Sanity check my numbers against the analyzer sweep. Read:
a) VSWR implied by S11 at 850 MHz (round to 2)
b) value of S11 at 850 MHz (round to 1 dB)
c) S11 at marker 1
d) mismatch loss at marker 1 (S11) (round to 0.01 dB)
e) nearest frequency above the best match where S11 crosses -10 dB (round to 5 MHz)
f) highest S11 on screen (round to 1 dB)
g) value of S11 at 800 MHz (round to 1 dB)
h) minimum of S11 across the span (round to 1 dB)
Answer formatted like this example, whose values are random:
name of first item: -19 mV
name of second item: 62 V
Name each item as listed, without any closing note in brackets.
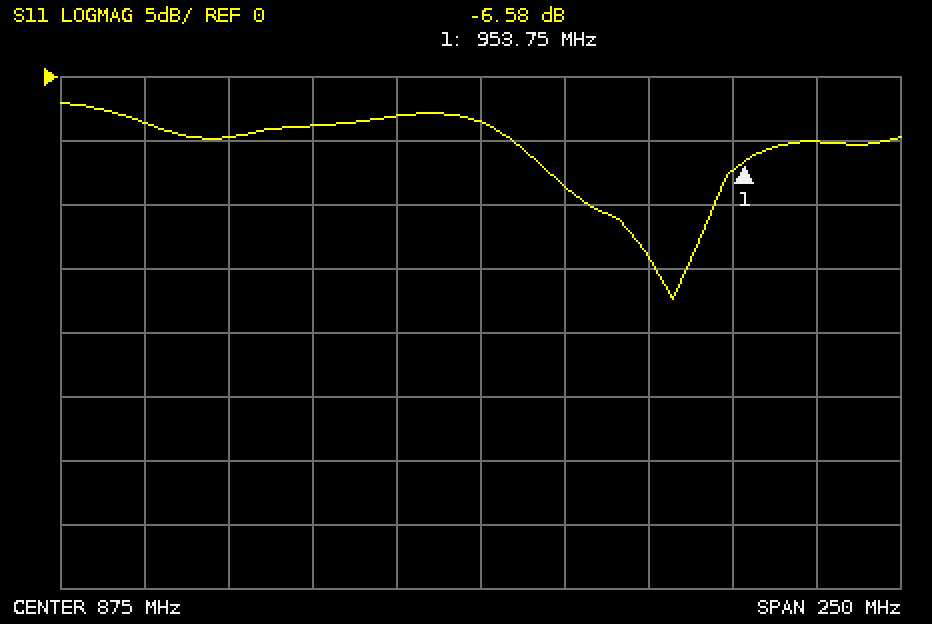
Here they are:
VSWR implied by S11 at 850 MHz: 6
value of S11 at 850 MHz: -3 dB
S11 at marker 1: -6.58 dB
mismatch loss at marker 1 (S11): 1.08 dB
nearest frequency above the best match where S11 crosses -10 dB: 945 MHz
highest S11 on screen: -2 dB
value of S11 at 800 MHz: -5 dB
minimum of S11 across the span: -17 dB
